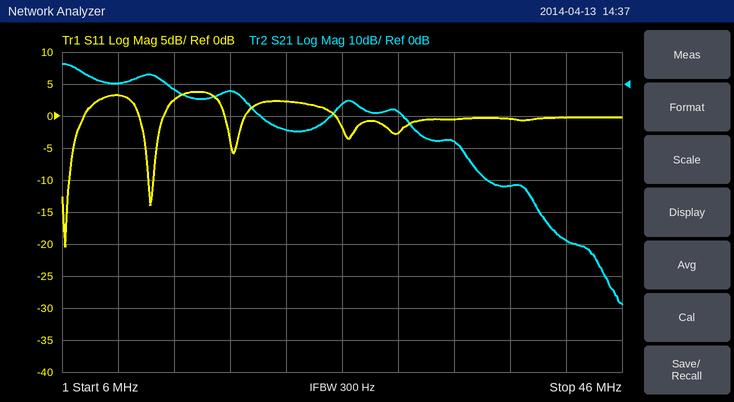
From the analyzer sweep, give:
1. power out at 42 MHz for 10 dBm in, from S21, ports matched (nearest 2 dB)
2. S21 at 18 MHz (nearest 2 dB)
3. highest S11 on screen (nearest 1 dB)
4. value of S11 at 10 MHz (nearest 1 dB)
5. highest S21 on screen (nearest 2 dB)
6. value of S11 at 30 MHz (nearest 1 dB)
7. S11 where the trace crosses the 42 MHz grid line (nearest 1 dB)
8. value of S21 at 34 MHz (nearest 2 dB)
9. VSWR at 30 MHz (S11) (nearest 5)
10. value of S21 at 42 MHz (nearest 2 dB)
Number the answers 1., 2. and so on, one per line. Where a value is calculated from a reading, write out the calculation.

1. 10 dBm + (-48 dB) = -38 dBm
2. -2 dB
3. 4 dB
4. 3 dB
5. 6 dB
6. -3 dB
7. 0 dB
8. -18 dB
9. |Γ| = 10^(-3/20) = 0.7079; VSWR = (1 + 0.7079)/(1 − 0.7079) ≈ 5.85, so 5 to the nearest 5
10. -48 dB
